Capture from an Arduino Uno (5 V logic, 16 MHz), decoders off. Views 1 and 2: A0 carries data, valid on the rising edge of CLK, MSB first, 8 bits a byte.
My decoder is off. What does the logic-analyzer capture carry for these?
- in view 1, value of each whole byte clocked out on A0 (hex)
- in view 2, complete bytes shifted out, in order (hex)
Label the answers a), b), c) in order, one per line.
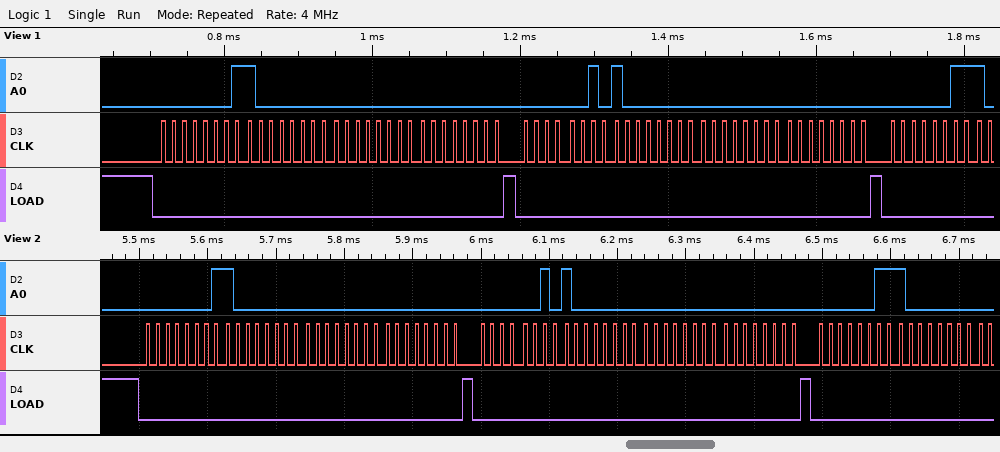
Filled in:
a) 01 80 00 00 02 80 00 00 03
b) 01 80 00 00 02 80 00 00 03 80
